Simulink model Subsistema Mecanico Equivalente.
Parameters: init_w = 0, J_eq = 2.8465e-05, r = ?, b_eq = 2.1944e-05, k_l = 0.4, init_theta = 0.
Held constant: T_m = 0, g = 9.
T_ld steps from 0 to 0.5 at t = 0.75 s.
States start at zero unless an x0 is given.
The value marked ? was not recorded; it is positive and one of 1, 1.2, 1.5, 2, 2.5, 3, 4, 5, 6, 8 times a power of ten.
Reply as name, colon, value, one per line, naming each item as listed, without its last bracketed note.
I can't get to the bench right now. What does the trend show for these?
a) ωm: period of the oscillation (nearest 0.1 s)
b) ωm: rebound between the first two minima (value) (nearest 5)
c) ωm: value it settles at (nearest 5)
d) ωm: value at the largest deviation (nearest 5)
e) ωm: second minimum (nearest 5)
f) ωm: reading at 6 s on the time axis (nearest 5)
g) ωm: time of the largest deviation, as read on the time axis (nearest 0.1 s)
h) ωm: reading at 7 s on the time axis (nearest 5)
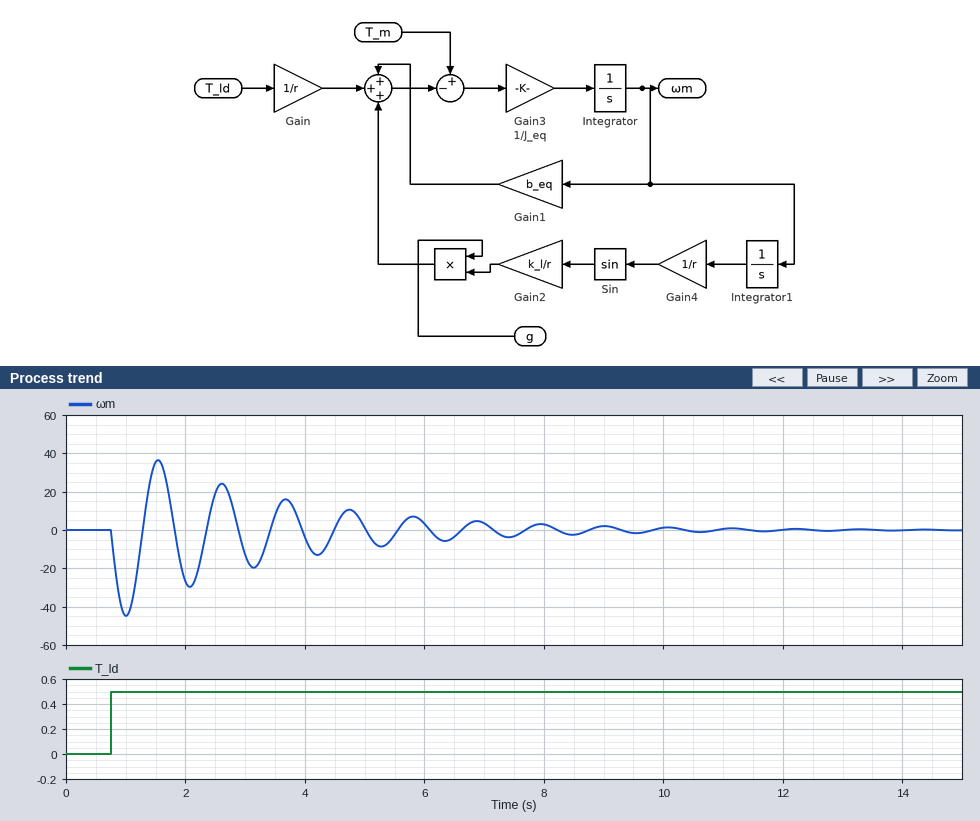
ωm: period of the oscillation: 1.1 s
ωm: rebound between the first two minima (value): 35
ωm: value it settles at: 0
ωm: value at the largest deviation: -45
ωm: second minimum: -30
ωm: reading at 6 s on the time axis: 5
ωm: time of the largest deviation, as read on the time axis: 1.0 s
ωm: reading at 7 s on the time axis: 5
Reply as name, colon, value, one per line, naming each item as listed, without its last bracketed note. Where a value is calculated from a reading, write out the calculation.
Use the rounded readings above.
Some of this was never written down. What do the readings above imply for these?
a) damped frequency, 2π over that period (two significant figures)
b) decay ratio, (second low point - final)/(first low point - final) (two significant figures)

damped frequency, 2π over that period: 2π / 1.1 = 5.7 rad/s
decay ratio, (second low point - final)/(first low point - final): (-30 - 0) / (-45 - 0) = 0.67
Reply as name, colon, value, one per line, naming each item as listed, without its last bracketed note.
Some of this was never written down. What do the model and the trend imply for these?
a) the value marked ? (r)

the value marked ?: 60
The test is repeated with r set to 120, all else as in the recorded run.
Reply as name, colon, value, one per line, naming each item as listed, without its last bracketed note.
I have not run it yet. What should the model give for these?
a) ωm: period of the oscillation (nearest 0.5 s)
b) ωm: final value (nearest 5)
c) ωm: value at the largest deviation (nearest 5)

ωm: period of the oscillation: 2.0 s
ωm: final value: 0
ωm: value at the largest deviation: -40
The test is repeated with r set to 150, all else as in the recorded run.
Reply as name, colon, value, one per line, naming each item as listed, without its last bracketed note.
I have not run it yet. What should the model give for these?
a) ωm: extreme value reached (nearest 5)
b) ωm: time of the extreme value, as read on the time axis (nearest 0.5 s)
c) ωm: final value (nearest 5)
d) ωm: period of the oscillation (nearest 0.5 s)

ωm: extreme value reached: -40
ωm: time of the extreme value, as read on the time axis: 1.5 s
ωm: final value: 0
ωm: period of the oscillation: 2.5 s
